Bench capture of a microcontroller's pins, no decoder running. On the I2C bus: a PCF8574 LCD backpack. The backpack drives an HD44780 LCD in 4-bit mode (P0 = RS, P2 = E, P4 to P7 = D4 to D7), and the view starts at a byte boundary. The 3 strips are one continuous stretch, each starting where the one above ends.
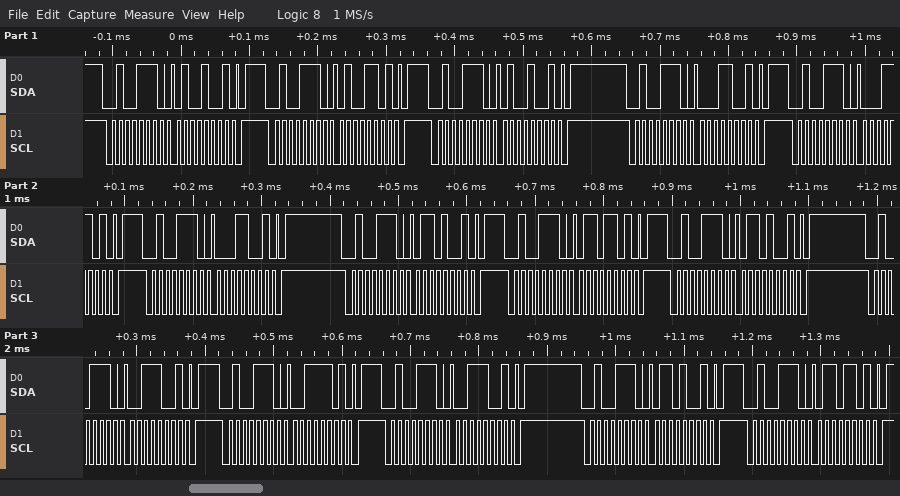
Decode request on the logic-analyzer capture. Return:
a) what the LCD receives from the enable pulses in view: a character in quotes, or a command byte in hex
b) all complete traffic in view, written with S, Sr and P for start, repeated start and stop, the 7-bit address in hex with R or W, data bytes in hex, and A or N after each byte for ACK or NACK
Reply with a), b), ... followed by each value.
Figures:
a) 'A' 'c'
b) S 27W A 49 A P S 27W A 4D A P S 27W A 49 A P S 27W A 19 A P S 27W A 1D A P S 27W A 19 A P S 27W A 69 A P S 27W A 6D A P S 27W A 69 A P S 27W A 39 A P S 27W A 3D A P S 27W A 39 A P S 27W A 69 A P S 27W A 6D A P
